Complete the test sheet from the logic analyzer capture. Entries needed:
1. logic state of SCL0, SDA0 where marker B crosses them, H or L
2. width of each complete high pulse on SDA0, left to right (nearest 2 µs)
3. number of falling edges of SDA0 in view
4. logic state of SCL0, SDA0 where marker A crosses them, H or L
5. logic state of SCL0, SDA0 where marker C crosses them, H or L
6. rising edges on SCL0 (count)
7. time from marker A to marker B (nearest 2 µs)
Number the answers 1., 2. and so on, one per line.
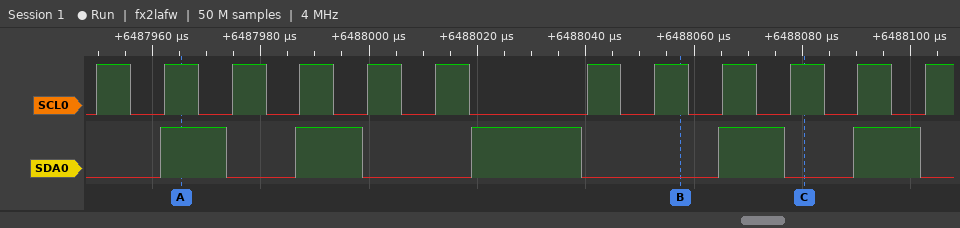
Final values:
1. SCL0=H, SDA0=L
2. 12 µs, 12 µs, 20 µs, 12 µs, 12 µs
3. 5
4. SCL0=H, SDA0=H
5. SCL0=H, SDA0=L
6. 12
7. 92 µs
